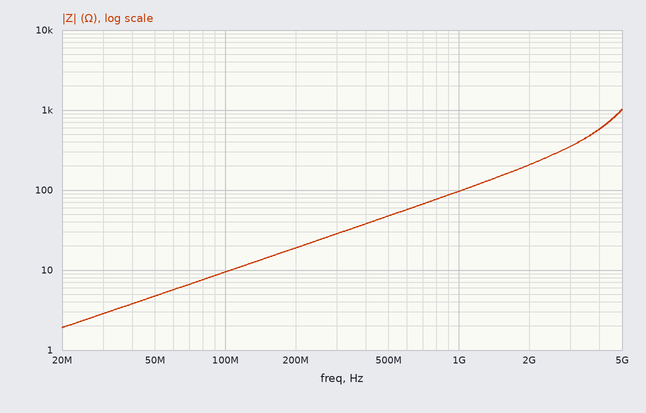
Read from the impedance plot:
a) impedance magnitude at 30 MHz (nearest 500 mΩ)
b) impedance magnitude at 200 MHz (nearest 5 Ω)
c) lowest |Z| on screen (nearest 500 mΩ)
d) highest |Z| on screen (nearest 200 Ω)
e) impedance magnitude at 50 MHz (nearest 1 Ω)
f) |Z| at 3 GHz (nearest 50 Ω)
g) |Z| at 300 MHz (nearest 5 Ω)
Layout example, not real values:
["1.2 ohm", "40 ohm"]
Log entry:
["3.0 Ω", "20 Ω", "2.0 Ω", "1.0 kΩ", "5 Ω", "350 Ω", "30 Ω"]
